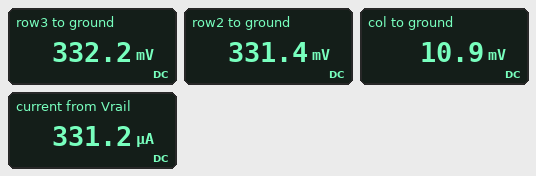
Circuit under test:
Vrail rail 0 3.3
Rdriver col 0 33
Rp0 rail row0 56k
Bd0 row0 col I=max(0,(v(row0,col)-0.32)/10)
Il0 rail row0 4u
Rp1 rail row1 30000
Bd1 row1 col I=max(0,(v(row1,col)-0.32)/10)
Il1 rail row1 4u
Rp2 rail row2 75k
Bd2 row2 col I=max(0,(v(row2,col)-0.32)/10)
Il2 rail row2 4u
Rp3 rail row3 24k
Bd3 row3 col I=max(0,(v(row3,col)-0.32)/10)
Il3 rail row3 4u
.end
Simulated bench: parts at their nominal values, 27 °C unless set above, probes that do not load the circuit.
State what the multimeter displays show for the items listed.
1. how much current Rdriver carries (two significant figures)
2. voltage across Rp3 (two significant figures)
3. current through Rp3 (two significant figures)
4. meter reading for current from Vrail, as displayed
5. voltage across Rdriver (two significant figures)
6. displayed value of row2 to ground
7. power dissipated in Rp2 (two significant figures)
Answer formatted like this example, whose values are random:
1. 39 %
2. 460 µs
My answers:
1. 330 µA
2. 3.0 V
3. 120 µA
4. 331.2 µA
5. 11 mV
6. 331.4 mV
7. 120 µW
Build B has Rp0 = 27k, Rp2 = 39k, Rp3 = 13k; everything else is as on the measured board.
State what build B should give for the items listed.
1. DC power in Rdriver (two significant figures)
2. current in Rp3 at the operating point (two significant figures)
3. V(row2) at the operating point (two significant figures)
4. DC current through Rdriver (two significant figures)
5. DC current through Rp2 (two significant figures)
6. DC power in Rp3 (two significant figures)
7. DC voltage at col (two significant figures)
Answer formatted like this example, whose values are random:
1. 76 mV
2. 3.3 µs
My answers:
1. 9.2 µW
2. 230 µA
3. 340 mV
4. 530 µA
5. 76 µA
6. 670 µW
7. 17 mV
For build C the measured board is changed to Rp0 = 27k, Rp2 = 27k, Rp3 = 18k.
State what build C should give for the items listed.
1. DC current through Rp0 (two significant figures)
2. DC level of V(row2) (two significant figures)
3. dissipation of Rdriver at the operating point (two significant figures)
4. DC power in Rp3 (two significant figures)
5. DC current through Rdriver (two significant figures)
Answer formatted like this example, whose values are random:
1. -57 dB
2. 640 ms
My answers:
1. 110 µA
2. 340 mV
3. 8.2 µW
4. 490 µW
5. 500 µA
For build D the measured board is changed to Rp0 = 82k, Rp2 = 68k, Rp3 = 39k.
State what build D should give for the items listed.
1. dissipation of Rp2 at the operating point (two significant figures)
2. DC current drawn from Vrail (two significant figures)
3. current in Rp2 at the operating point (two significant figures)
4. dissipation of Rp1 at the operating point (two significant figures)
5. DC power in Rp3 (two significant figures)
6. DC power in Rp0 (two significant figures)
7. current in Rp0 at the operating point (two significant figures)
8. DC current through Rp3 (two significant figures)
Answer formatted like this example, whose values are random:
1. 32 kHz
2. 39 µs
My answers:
1. 130 µW
2. 270 µA
3. 44 µA
4. 290 µW
5. 230 µW
6. 110 µW
7. 36 µA
8. 76 µA
